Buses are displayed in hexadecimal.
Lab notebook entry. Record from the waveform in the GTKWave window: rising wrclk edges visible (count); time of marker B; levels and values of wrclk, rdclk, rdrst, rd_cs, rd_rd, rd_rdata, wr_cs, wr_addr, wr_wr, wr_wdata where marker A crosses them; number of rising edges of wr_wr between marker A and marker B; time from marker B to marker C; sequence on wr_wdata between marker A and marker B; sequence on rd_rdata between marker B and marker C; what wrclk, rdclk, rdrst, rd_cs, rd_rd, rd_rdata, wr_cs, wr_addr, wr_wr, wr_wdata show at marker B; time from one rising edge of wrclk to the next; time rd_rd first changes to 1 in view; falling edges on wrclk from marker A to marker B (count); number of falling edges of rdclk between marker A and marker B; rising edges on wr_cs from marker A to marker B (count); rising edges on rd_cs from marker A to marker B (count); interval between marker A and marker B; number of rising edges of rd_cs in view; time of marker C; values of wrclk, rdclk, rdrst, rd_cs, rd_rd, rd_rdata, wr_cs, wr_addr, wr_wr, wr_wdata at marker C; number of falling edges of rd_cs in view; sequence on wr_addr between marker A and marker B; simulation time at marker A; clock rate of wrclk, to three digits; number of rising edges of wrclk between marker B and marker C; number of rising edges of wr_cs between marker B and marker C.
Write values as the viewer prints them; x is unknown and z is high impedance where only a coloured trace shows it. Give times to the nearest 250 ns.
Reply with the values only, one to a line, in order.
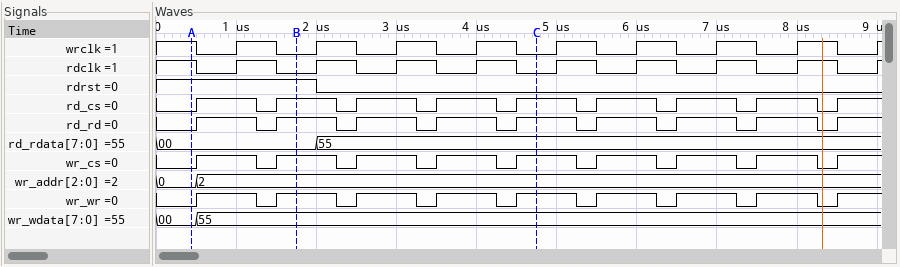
9
1750 ns
wrclk=1, rdclk=1, rdrst=1, rd_cs=0, rd_rd=0, rd_rdata=00, wr_cs=0, wr_addr=0, wr_wr=0, wr_wdata=00
2
3000 ns
00, 55
00, 55
wrclk=0, rdclk=0, rdrst=1, rd_cs=1, rd_rd=1, rd_rdata=00, wr_cs=1, wr_addr=2, wr_wr=1, wr_wdata=55
1000 ns
500 ns
2
2
2
2
1250 ns
9
4750 ns
wrclk=0, rdclk=0, rdrst=0, rd_cs=1, rd_rd=1, rd_rdata=55, wr_cs=1, wr_addr=2, wr_wr=1, wr_wdata=55
8
0, 2
500 ns
1.00 MHz
3
3
